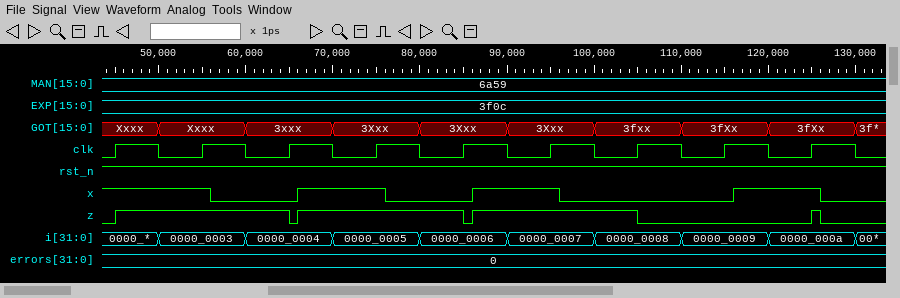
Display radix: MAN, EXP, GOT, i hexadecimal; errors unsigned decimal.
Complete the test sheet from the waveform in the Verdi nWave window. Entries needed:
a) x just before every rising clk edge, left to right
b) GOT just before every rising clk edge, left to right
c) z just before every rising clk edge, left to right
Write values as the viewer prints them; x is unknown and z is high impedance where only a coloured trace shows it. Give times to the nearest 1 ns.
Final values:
1 1 0 1 0 1 0 0 1
Xxxx, Xxxx, 3xxx, 3Xxx, 3Xxx, 3Xxx, 3fxx, 3fXx, 3fXx
0 1 1 1 1 1 1 0 0
